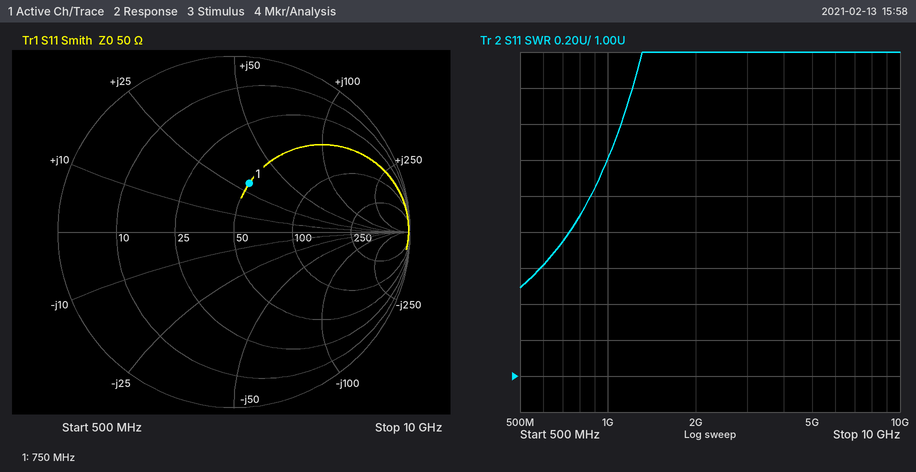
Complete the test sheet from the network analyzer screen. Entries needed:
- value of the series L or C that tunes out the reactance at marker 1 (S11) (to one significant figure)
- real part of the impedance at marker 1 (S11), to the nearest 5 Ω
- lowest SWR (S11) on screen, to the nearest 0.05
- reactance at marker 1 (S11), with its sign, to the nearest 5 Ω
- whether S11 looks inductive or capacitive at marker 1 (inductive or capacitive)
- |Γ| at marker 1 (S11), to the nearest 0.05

7 pF
50 Ω
1.50
+30 Ω
inductive
0.30
